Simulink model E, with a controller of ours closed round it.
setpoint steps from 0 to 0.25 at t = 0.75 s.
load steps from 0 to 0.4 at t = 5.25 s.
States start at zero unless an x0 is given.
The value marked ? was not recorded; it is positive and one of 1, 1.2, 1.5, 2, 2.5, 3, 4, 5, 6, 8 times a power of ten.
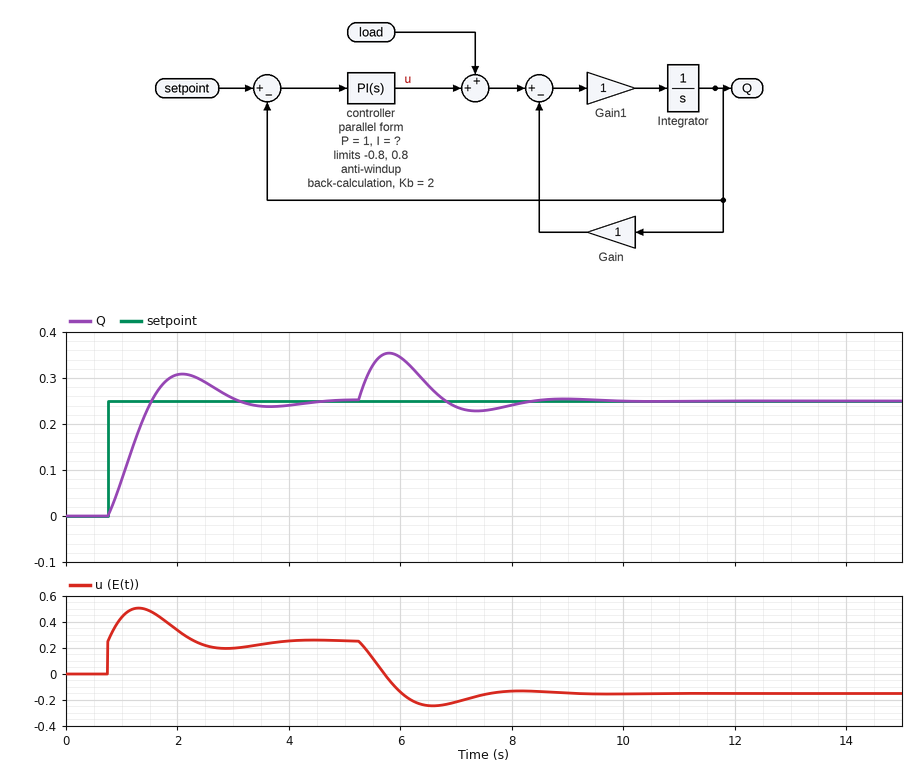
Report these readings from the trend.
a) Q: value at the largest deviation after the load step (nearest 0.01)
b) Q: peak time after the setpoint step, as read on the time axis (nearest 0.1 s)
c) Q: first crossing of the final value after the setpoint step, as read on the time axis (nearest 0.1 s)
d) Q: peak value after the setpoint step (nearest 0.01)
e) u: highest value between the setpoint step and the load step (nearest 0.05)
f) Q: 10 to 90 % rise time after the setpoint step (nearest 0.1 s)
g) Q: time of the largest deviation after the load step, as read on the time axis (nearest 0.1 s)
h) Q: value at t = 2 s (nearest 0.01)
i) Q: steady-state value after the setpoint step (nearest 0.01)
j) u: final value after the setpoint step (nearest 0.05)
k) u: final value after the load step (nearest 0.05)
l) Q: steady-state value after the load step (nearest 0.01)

0.35
2.1 s
1.5 s
0.31
0.50
0.6 s
5.8 s
0.31
0.25
0.25
-0.15
0.25
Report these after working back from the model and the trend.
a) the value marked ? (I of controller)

5
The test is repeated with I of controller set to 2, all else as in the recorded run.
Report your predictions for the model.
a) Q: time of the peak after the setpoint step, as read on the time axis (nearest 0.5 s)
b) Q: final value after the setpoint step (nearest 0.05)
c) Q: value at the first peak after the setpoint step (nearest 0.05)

3.0 s
0.25
0.25
